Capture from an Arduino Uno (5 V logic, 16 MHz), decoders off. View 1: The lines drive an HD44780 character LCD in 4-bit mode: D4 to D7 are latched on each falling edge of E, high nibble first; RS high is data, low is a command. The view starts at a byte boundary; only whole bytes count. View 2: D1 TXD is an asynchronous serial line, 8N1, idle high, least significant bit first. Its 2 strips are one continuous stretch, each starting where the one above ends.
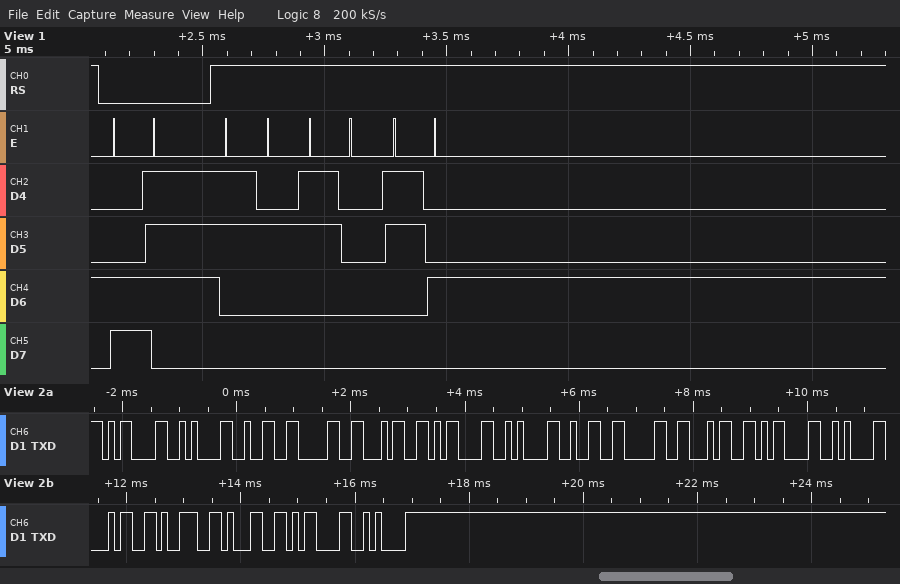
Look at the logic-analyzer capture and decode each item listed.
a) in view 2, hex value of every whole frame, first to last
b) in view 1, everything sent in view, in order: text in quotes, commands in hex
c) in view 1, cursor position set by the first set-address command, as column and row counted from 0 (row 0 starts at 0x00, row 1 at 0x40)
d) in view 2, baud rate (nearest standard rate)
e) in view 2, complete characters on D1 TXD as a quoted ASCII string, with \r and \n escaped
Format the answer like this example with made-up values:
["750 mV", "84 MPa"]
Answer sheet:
["0D 0A 32 30 34 0D 0A 32 30 34 0D 0A 34 39 31 0D 0A", "0xC7 \"204\"", "column 7, row 1", "9600 baud", "\"\\r\\n204\\r\\n204\\r\\n491\\r\\n\""]
